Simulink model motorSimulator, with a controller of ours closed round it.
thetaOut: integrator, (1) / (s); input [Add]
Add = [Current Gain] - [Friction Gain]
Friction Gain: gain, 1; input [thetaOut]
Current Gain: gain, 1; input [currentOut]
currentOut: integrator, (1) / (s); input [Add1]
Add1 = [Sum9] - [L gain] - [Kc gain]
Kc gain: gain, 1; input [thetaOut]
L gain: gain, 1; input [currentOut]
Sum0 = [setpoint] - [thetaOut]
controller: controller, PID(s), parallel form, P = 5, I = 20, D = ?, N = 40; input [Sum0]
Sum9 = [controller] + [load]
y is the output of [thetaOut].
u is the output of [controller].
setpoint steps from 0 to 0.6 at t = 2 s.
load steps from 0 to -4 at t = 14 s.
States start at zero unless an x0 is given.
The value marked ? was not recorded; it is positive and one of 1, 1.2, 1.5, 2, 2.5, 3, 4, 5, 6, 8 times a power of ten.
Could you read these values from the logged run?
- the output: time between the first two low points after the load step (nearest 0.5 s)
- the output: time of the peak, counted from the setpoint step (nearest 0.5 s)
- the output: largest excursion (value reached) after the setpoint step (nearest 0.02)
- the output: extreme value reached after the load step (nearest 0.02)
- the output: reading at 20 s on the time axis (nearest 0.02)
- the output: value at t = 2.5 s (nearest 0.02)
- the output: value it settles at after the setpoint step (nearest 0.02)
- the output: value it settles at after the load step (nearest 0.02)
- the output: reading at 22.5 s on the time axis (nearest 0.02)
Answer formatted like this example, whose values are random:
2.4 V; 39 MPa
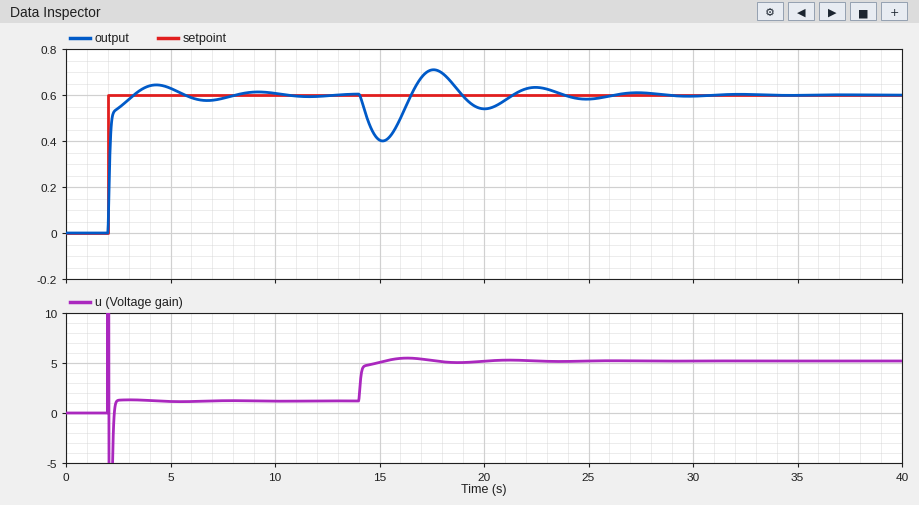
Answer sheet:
5.0 s; 2.5 s; 0.64; 0.40; 0.54; 0.54; 0.60; 0.60; 0.64
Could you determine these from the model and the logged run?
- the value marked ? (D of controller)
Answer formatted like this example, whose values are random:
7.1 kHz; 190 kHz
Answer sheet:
10
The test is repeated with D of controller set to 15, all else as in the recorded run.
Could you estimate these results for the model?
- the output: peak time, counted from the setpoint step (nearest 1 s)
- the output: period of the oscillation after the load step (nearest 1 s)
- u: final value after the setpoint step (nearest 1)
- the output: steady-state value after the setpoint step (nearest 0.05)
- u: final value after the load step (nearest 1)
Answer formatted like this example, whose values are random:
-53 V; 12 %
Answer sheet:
3 s; 6 s; 1; 0.60; 5
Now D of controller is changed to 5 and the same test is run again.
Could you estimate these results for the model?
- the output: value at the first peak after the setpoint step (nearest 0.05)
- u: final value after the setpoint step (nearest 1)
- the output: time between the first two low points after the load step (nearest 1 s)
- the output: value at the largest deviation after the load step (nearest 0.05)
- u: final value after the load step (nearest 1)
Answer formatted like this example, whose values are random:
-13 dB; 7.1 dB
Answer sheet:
0.70; 1; 4 s; 0.35; 5
